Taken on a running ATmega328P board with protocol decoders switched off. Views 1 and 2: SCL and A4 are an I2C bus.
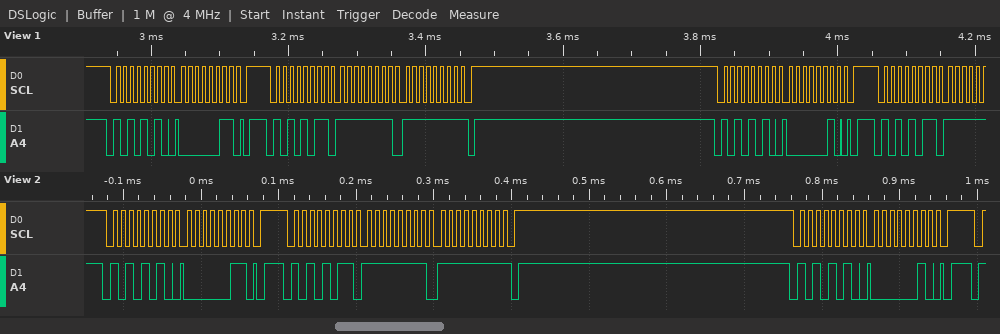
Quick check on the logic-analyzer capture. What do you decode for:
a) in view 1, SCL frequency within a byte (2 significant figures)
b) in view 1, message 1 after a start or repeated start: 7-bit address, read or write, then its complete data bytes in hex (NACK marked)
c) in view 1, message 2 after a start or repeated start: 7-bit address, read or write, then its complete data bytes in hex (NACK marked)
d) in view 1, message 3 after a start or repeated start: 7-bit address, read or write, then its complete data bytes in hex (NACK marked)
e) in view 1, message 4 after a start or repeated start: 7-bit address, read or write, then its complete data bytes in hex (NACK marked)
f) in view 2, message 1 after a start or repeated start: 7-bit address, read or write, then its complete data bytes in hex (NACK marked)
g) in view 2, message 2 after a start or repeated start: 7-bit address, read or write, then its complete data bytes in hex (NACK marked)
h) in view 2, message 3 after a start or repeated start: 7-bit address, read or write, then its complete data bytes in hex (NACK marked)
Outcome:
100 kHz
0x55 write: 03
0x55 read: FF FF NACK
0x55 write: 02
0x55 read
0x55 write: 03
0x55 read: FF FF NACK
0x55 write: 02
